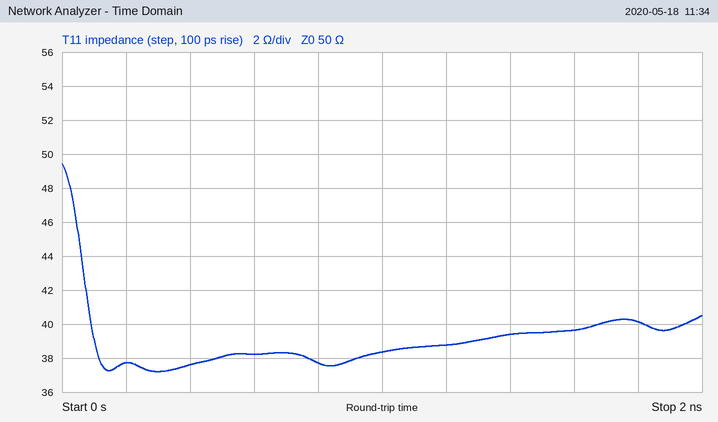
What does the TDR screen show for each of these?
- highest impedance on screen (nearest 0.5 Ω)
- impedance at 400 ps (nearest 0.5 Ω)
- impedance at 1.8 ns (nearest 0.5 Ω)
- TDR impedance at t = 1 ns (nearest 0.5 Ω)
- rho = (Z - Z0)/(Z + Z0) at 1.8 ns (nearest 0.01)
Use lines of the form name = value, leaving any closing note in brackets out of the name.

highest impedance on screen = 49.5 Ω
impedance at 400 ps = 37.5 Ω
impedance at 1.8 ns = 40.0 Ω
TDR impedance at t = 1 ns = 38.5 Ω
rho = (Z - Z0)/(Z + Z0) at 1.8 ns = -0.11
